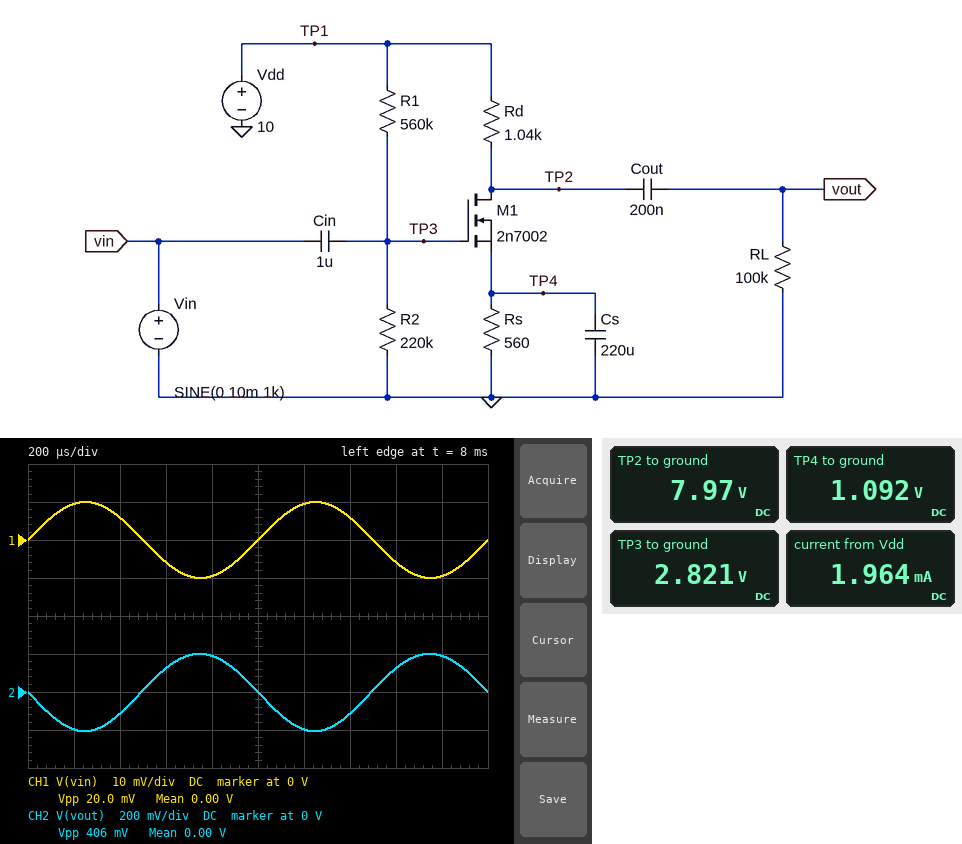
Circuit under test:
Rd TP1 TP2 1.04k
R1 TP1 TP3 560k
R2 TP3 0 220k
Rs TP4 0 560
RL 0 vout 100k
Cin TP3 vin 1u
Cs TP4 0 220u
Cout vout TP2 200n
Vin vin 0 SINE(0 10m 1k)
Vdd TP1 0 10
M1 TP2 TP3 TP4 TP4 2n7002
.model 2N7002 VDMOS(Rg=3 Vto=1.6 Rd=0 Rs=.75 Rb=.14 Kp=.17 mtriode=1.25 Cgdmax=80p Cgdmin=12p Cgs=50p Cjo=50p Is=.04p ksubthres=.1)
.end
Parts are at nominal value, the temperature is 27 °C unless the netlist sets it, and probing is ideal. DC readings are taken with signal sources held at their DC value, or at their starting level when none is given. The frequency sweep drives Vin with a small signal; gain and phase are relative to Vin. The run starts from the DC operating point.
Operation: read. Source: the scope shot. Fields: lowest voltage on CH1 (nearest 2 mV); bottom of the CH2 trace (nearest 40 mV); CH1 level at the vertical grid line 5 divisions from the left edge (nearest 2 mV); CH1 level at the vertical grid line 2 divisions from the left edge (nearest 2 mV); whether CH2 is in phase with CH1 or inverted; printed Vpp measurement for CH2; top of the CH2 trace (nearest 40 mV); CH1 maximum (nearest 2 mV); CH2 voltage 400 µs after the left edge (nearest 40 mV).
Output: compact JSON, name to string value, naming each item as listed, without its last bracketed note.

{"lowest voltage on CH1": "-10 mV", "bottom of the CH2 trace": "-200 mV", "CH1 level at the vertical grid line 5 divisions from the left edge": "0 V", "CH1 level at the vertical grid line 2 divisions from the left edge": "6 mV", "whether CH2 is in phase with CH1 or inverted": "inverted", "printed Vpp measurement for CH2": "406 mV", "top of the CH2 trace": "200 mV", "CH1 maximum": "10 mV", "CH2 voltage 400 µs after the left edge": "-120 mV"}
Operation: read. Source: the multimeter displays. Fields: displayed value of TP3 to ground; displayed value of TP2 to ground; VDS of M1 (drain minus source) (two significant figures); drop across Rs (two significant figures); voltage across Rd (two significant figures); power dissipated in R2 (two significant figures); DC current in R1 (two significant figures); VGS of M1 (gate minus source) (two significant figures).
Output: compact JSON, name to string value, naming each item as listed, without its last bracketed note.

{"displayed value of TP3 to ground": "2.821 V", "displayed value of TP2 to ground": "7.97 V", "VDS of M1 (drain minus source)": "6.9 V", "drop across Rs": "1.1 V", "voltage across Rd": "2.0 V", "power dissipated in R2": "36 µW", "DC current in R1": "13 µA", "VGS of M1 (gate minus source)": "1.7 V"}
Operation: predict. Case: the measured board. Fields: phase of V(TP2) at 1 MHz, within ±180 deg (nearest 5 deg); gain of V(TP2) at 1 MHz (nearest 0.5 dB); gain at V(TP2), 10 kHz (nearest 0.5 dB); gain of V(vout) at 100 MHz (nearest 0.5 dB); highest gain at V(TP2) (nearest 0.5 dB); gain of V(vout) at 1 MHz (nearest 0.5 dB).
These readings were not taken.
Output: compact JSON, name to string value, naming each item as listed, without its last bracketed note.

{"phase of V(TP2) at 1 MHz, within ±180 deg": "165 deg", "gain of V(TP2) at 1 MHz": "26.0 dB", "gain at V(TP2), 10 kHz": "26.0 dB", "gain of V(vout) at 100 MHz": "0.5 dB", "highest gain at V(TP2)": "26.0 dB", "gain of V(vout) at 1 MHz": "26.0 dB"}
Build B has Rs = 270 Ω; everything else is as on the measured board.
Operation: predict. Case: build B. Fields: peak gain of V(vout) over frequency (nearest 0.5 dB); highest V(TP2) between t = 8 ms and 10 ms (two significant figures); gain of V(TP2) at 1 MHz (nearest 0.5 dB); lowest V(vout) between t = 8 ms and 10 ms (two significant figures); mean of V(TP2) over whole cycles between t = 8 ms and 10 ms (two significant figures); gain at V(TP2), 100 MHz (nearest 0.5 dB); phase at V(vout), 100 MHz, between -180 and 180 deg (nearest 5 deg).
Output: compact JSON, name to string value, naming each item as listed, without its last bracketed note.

{"peak gain of V(vout) over frequency": "30.0 dB", "highest V(TP2) between t = 8 ms and 10 ms": "6.4 V", "gain of V(TP2) at 1 MHz": "29.5 dB", "lowest V(vout) between t = 8 ms and 10 ms": "-320 mV", "mean of V(TP2) over whole cycles between t = 8 ms and 10 ms": "6.1 V", "gain at V(TP2), 100 MHz": "2.5 dB", "phase at V(vout), 100 MHz, between -180 and 180 deg": "65 deg"}
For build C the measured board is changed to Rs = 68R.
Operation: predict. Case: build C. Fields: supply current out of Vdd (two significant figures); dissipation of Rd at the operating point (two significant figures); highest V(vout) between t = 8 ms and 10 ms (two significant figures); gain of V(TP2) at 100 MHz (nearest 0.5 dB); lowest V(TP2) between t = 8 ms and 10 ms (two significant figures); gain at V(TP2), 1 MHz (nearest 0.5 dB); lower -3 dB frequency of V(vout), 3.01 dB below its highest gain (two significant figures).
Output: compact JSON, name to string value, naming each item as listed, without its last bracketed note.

{"supply current out of Vdd": "9.0 mA", "dissipation of Rd at the operating point": "83 mW", "highest V(vout) between t = 8 ms and 10 ms": "1.5 mV", "gain of V(TP2) at 100 MHz": "-8.0 dB", "lowest V(TP2) between t = 8 ms and 10 ms": "690 mV", "gain at V(TP2), 1 MHz": "-16.5 dB", "lower -3 dB frequency of V(vout), 3.01 dB below its highest gain": "77 MHz"}
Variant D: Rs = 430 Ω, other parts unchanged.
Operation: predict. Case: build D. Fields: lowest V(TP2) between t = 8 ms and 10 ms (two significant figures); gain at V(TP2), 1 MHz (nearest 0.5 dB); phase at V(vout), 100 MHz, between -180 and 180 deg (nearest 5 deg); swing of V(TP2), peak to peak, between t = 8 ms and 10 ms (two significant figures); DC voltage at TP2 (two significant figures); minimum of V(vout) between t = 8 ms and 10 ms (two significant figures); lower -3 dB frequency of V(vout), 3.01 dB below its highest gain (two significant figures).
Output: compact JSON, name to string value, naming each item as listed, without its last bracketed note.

{"lowest V(TP2) between t = 8 ms and 10 ms": "7.2 V", "gain at V(TP2), 1 MHz": "27.5 dB", "phase at V(vout), 100 MHz, between -180 and 180 deg": "60 deg", "swing of V(TP2), peak to peak, between t = 8 ms and 10 ms": "480 mV", "DC voltage at TP2": "7.4 V", "minimum of V(vout) between t = 8 ms and 10 ms": "-240 mV", "lower -3 dB frequency of V(vout), 3.01 dB below its highest gain": "21 Hz"}
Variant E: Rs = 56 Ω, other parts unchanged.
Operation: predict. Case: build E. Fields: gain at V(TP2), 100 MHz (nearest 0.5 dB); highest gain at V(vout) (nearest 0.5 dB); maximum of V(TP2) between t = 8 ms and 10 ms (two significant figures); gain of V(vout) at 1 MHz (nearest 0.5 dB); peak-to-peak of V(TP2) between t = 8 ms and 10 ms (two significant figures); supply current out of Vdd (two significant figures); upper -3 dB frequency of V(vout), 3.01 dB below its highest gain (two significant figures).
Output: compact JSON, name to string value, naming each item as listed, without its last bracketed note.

{"gain at V(TP2), 100 MHz": "-9.0 dB", "highest gain at V(vout)": "-6.5 dB", "maximum of V(TP2) between t = 8 ms and 10 ms": "580 mV", "gain of V(vout) at 1 MHz": "-20.0 dB", "peak-to-peak of V(TP2) between t = 8 ms and 10 ms": "2.0 mV", "supply current out of Vdd": "9.1 mA", "upper -3 dB frequency of V(vout), 3.01 dB below its highest gain": "1.0 GHz"}
